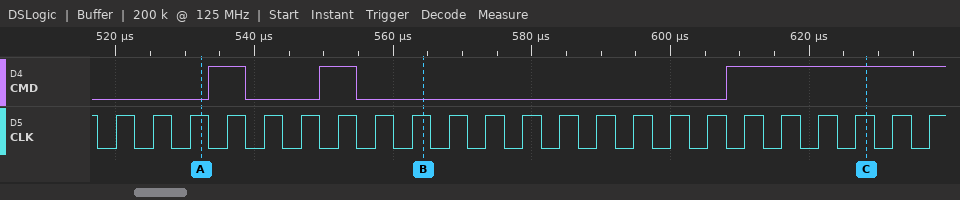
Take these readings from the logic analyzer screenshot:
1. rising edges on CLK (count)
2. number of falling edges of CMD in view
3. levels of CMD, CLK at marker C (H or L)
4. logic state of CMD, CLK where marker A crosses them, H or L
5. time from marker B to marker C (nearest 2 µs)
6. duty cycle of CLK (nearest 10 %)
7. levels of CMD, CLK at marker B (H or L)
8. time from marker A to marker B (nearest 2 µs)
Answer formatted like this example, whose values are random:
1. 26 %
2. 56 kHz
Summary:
1. 23
2. 2
3. CMD=H, CLK=H
4. CMD=L, CLK=H
5. 64 µs
6. 50 %
7. CMD=L, CLK=H
8. 32 µs
